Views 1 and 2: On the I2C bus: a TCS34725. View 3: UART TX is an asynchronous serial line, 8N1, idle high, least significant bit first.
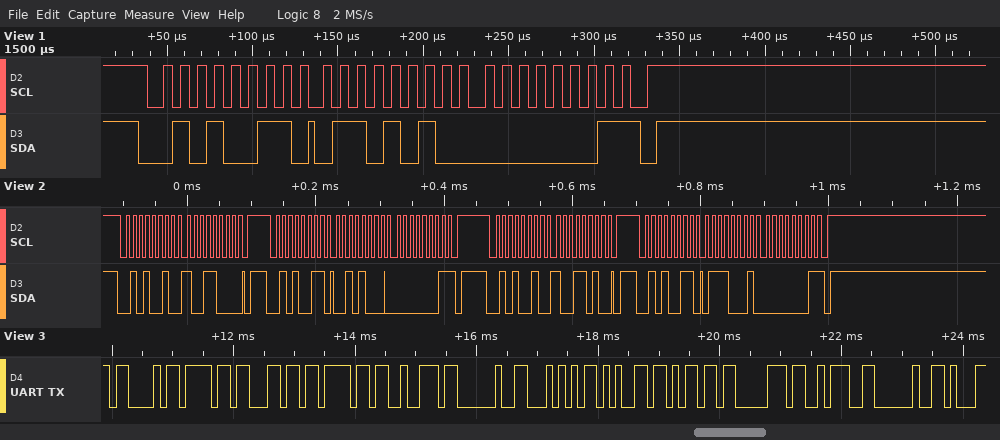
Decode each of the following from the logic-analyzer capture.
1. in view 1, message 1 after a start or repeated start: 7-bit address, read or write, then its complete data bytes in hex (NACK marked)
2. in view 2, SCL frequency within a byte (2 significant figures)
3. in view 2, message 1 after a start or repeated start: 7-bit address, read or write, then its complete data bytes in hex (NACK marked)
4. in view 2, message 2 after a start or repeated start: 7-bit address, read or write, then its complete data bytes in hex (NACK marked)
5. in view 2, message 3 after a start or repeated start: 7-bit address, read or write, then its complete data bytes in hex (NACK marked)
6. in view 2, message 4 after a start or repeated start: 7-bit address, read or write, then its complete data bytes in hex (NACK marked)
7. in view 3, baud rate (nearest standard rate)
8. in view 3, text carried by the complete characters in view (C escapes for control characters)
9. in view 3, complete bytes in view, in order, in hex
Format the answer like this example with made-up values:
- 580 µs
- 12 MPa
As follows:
- 0x29 read: 6A 01 NACK
- 100 kHz
- 0x29 write: 98
- 0x29 read: 28 01 NACK
- 0x29 write: 9A
- 0x29 read: 71 01 NACK
- 9600 baud
- "Color Temp: "
- 43 6F 6C 6F 72 20 54 65 6D 70 3A 20
